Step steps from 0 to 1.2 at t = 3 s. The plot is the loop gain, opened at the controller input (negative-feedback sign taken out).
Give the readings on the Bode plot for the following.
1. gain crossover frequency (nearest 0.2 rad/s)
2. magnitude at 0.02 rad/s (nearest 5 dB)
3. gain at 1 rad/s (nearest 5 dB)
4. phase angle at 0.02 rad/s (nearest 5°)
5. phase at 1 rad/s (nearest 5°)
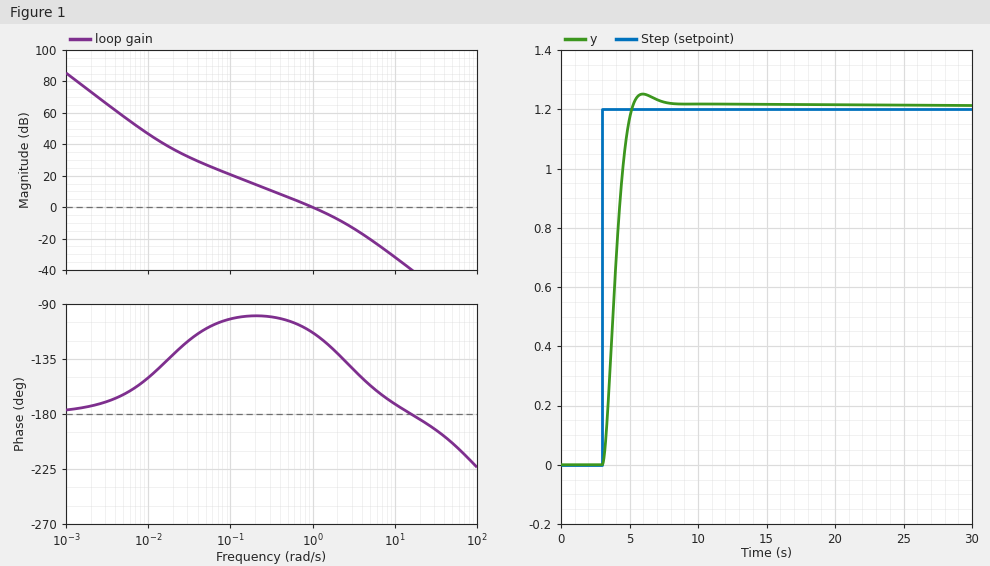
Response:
1.0 rad/s
35 dB
0 dB
-130°
-115°
